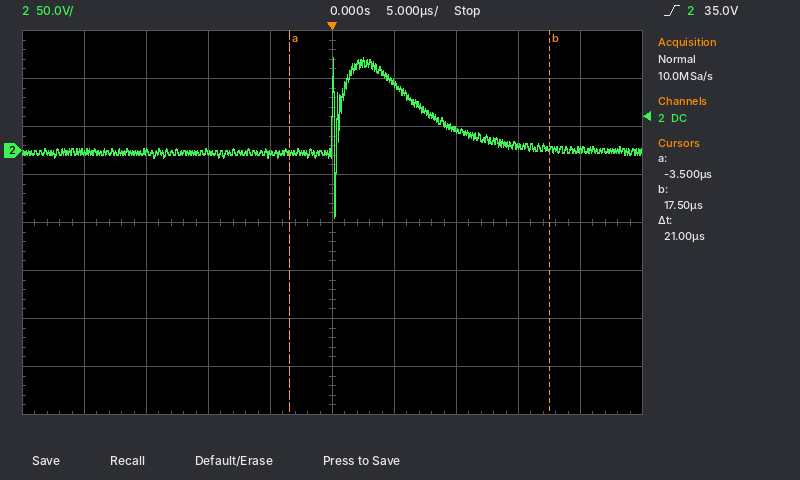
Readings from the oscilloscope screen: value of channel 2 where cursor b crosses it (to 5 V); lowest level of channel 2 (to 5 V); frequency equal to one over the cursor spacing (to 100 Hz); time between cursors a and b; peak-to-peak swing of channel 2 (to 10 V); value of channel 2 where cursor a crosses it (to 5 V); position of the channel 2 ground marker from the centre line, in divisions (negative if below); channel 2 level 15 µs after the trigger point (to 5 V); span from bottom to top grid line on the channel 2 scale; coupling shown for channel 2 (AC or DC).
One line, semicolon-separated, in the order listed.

0 V; -70 V; 47.6 kHz; 21 µs; 170 V; 0 V; +1.5 div; 5 V; 400 V; DC
